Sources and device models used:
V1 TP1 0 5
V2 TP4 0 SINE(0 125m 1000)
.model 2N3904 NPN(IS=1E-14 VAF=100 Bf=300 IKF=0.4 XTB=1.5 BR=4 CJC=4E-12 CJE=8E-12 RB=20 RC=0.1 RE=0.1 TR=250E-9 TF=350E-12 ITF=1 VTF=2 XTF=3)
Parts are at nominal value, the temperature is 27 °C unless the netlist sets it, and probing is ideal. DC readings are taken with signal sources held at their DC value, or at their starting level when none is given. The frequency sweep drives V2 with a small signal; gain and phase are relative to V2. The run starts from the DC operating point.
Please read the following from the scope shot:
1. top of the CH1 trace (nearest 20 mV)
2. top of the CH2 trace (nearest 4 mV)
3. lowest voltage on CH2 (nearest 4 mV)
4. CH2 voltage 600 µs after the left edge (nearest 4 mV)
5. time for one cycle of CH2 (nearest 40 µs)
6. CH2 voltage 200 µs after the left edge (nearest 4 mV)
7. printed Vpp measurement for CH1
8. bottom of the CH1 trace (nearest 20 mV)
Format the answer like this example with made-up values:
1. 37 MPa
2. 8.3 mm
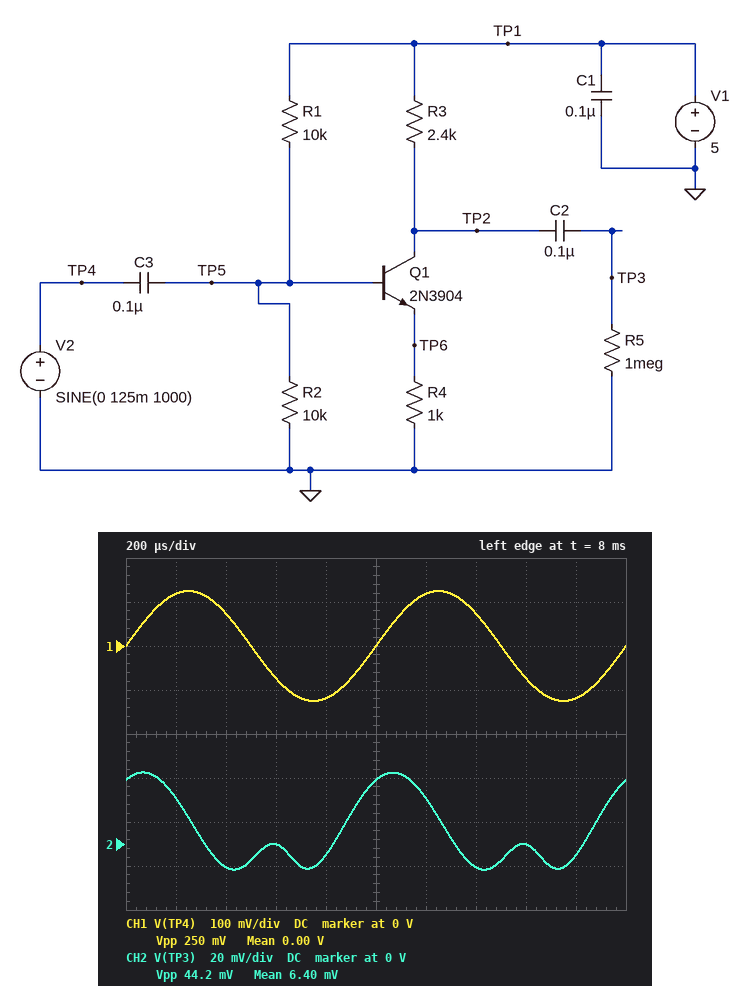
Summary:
1. 120 mV
2. 32 mV
3. -12 mV
4. 0 V
5. 1.00 ms
6. 20 mV
7. 250 mV
8. -120 mV
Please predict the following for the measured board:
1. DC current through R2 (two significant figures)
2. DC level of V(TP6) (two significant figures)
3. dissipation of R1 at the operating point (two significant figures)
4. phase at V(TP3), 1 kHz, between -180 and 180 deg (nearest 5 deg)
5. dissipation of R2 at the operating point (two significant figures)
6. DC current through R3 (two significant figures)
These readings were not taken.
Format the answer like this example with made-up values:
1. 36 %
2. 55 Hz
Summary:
1. 220 µA
2. 1.5 V
3. 800 µW
4. 65 deg
5. 470 µW
6. 1.4 mA
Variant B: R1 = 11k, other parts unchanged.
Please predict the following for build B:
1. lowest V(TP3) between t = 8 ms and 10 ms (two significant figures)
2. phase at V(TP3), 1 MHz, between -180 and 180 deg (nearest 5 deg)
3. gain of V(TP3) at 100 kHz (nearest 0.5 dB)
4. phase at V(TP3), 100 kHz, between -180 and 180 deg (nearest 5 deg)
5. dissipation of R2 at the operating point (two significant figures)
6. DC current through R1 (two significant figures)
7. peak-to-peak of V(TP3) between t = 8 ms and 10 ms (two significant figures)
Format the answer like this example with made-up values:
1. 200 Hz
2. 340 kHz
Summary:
1. -5.1 mV
2. 10 deg
3. -6.0 dB
4. 35 deg
5. 460 µW
6. 260 µA
7. 93 mV
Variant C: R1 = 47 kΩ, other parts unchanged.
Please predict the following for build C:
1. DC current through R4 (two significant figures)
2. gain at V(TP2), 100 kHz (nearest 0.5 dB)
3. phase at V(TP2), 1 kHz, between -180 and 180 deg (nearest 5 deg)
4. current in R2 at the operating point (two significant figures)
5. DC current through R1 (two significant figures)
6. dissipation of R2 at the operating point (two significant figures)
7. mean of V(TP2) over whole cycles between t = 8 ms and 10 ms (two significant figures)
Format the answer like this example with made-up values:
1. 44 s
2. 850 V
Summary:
1. 250 µA
2. 6.5 dB
3. -170 deg
4. 87 µA
5. 88 µA
6. 76 µW
7. 4.4 V
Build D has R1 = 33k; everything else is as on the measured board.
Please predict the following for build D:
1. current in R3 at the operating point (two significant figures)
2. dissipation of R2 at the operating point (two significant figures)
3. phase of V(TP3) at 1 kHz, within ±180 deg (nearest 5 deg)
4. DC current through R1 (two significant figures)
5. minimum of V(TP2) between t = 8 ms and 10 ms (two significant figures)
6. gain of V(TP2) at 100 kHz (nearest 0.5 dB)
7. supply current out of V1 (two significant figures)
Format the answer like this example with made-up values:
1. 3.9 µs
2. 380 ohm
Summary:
1. 510 µA
2. 130 µW
3. -170 deg
4. 120 µA
5. 3.5 V
6. 7.0 dB
7. 630 µA
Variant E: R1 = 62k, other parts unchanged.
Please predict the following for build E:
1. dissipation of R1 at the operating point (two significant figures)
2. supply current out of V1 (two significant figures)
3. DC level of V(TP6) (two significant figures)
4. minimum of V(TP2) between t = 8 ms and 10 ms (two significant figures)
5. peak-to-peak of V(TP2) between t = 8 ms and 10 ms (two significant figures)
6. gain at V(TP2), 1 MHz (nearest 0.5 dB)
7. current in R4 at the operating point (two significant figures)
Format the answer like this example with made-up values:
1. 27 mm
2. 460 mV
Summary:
1. 300 µW
2. 170 µA
3. 98 mV
4. 4.5 V
5. 440 mV
6. 5.5 dB
7. 98 µA
